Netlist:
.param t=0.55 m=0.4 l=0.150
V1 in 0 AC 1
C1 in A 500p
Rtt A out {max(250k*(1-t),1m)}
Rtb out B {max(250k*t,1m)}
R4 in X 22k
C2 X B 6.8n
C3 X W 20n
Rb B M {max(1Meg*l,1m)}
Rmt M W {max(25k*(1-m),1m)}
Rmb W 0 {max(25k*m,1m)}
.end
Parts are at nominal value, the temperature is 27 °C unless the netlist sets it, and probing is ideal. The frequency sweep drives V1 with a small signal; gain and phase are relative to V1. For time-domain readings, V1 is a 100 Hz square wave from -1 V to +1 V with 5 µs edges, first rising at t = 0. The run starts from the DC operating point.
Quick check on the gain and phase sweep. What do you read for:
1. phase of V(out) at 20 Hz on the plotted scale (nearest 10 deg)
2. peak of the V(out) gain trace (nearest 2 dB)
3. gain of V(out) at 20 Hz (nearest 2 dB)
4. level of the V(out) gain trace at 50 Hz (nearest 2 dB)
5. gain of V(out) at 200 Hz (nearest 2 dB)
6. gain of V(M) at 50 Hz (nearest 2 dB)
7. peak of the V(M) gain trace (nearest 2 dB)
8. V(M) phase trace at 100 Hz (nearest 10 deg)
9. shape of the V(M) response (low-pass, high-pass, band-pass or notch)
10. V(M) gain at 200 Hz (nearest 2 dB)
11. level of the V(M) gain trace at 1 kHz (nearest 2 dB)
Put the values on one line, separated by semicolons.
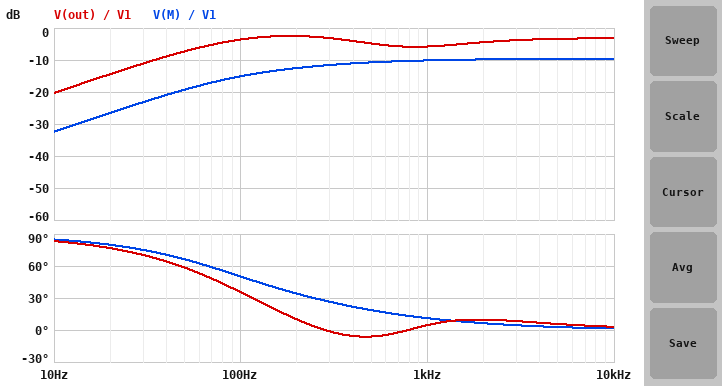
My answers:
80 deg; -2 dB; -14 dB; -8 dB; -2 dB; -20 dB; -10 dB; 50 deg; high-pass; -12 dB; -10 dB
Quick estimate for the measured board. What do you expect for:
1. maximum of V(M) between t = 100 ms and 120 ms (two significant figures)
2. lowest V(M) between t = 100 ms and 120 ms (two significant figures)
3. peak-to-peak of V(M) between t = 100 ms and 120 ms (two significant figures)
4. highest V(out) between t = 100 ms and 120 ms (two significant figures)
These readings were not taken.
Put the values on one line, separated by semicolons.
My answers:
640 mV; -640 mV; 1.3 V; 1.3 V
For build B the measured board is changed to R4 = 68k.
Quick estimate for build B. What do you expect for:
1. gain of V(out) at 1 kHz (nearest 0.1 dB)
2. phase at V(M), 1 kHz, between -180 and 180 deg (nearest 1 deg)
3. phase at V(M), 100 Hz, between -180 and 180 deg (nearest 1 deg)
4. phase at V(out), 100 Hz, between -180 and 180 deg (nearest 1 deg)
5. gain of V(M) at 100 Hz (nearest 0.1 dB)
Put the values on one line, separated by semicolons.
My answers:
-8.3 dB; 7 deg; 30 deg; 19 deg; -18.1 dB
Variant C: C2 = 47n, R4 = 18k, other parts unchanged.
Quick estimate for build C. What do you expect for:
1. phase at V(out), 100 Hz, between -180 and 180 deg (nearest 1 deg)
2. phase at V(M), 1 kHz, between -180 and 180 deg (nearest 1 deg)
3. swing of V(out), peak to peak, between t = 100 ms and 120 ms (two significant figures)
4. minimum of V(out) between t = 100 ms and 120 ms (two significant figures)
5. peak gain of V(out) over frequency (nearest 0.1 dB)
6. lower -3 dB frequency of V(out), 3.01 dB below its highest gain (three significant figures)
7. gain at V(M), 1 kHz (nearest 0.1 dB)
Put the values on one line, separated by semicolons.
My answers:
0 deg; 13 deg; 1.9 V; -970 mV; -1.1 dB; 15.7 Hz; -9.2 dB
